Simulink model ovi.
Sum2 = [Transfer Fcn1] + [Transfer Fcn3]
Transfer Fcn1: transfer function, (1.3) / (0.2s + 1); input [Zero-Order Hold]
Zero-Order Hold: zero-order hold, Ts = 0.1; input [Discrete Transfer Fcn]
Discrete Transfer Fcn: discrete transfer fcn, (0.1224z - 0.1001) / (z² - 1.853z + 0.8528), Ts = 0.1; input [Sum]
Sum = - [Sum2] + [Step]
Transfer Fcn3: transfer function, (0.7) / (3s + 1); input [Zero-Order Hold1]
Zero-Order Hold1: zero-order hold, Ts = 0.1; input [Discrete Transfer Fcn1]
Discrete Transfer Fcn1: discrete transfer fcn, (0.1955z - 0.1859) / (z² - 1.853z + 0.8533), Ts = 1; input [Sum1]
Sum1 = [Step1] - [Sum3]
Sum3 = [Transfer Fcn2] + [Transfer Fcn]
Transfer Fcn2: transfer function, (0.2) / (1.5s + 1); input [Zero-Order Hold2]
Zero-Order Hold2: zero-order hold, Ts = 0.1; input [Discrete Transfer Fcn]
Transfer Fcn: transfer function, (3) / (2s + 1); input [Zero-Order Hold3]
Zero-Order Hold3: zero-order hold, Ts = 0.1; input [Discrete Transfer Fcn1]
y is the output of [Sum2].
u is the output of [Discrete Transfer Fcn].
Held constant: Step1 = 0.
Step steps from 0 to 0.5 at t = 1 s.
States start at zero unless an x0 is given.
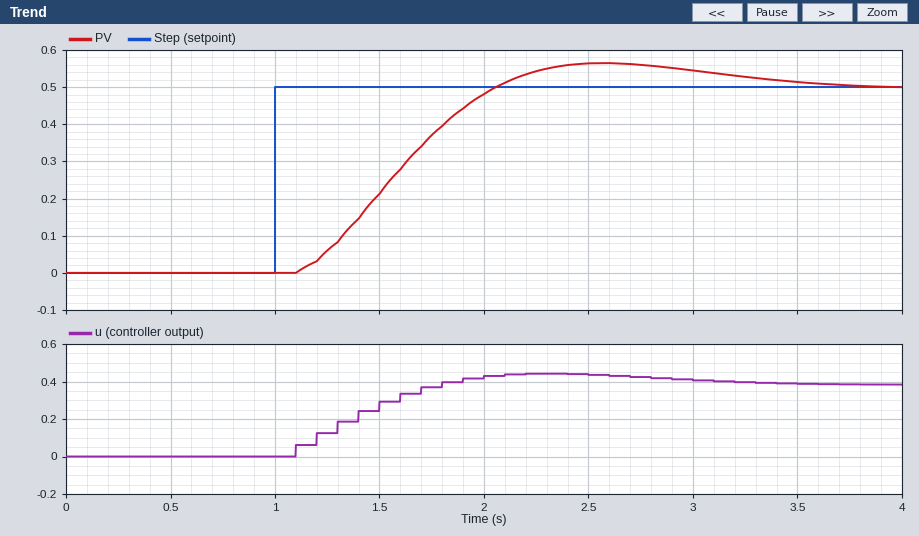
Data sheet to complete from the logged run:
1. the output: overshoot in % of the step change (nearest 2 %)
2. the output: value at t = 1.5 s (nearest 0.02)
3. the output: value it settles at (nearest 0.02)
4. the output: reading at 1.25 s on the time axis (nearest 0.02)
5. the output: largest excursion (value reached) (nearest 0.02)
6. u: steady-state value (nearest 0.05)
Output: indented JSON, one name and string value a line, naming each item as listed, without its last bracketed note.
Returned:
{
  "the output: overshoot in % of the step change": "12 %",
  "the output: value at t = 1.5 s": "0.22",
  "the output: value it settles at": "0.50",
  "the output: reading at 1.25 s on the time axis": "0.06",
  "the output: largest excursion (value reached)": "0.56",
  "u: steady-state value": "0.40"
}
